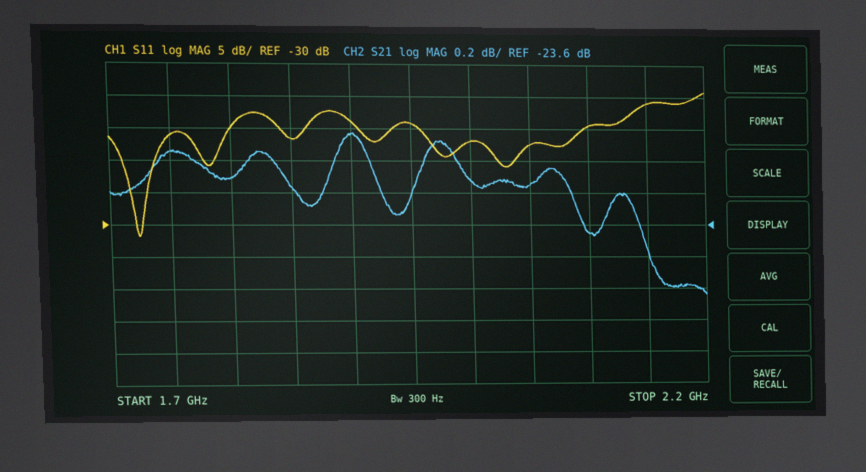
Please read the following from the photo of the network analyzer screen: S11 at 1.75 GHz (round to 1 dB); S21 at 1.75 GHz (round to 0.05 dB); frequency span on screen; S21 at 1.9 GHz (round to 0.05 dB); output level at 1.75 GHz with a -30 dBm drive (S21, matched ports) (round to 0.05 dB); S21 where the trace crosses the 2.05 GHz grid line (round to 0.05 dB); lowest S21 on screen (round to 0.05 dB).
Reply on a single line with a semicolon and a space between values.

-16 dB; -23.15 dB; 500 MHz; -23.05 dB; -53.15 dBm; -23.35 dB; -24.05 dB
